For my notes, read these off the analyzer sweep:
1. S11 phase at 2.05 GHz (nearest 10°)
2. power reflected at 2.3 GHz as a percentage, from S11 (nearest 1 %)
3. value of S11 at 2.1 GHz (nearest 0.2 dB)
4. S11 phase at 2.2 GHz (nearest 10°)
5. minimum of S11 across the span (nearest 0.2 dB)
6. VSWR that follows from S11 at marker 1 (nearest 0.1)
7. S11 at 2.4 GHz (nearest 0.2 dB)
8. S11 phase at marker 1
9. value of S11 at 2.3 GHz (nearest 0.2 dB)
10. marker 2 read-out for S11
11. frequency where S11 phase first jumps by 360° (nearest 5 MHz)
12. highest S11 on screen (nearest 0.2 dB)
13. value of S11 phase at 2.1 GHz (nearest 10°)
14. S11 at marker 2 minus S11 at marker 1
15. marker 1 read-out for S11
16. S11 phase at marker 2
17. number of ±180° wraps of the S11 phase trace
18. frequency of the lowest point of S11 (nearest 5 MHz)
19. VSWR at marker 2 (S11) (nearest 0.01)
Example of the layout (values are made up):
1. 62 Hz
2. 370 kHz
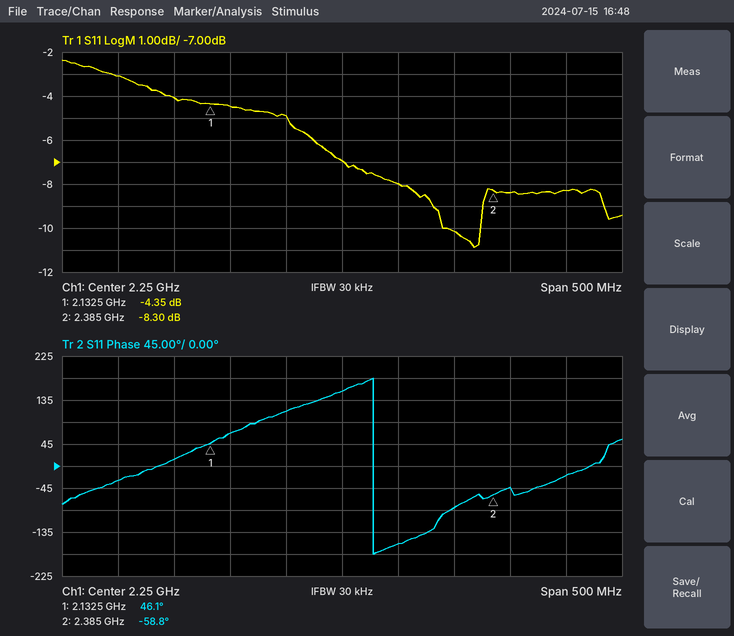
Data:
1. -30°
2. 16 %
3. -4.0 dB
4. 110°
5. -10.8 dB
6. 4.1
7. -8.4 dB
8. 46.1°
9. -8.0 dB
10. -8.30 dB
11. 2.280 GHz
12. -2.4 dB
13. 10°
14. -3.95 dB
15. -4.35 dB
16. -58.8°
17. 1
18. 2.370 GHz
19. 2.25
